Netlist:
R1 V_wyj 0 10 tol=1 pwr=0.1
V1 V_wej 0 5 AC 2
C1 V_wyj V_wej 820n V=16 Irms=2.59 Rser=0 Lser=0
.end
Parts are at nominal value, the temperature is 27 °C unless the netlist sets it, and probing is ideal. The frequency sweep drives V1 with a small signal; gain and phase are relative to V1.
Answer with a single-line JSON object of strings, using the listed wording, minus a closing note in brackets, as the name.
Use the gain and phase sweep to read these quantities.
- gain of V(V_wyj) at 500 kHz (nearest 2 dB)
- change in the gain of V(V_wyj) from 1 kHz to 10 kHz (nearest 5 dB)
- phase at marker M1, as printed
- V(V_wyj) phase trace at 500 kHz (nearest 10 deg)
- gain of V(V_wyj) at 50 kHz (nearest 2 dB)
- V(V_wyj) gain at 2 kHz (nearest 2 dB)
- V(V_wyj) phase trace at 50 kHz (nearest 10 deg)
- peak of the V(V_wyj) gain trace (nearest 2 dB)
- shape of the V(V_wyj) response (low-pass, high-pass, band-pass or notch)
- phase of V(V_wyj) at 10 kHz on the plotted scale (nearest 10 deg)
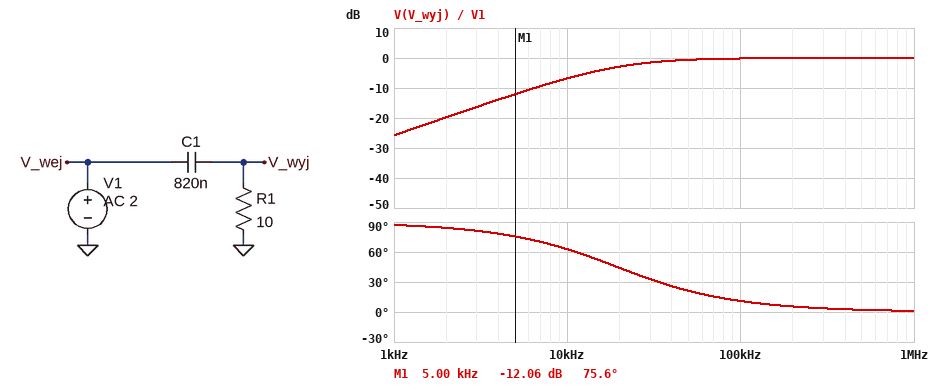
{"gain of V(V_wyj) at 500 kHz": "0 dB", "change in the gain of V(V_wyj) from 1 kHz to 10 kHz": "20 dB", "phase at marker M1, as printed": "75.6 deg", "V(V_wyj) phase trace at 500 kHz": "0 deg", "gain of V(V_wyj) at 50 kHz": "0 dB", "V(V_wyj) gain at 2 kHz": "-20 dB", "V(V_wyj) phase trace at 50 kHz": "20 deg", "peak of the V(V_wyj) gain trace": "0 dB", "shape of the V(V_wyj) response": "high-pass", "phase of V(V_wyj) at 10 kHz on the plotted scale": "60 deg"}
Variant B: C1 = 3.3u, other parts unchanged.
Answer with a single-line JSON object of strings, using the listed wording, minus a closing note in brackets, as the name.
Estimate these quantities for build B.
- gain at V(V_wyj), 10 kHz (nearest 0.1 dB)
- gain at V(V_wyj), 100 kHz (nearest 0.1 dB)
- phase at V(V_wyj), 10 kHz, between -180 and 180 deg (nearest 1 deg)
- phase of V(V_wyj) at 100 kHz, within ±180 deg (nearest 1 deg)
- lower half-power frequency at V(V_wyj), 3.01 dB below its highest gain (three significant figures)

{"gain at V(V_wyj), 10 kHz": "-0.9 dB", "gain at V(V_wyj), 100 kHz": "0 dB", "phase at V(V_wyj), 10 kHz, between -180 and 180 deg": "26 deg", "phase of V(V_wyj) at 100 kHz, within ±180 deg": "3 deg", "lower half-power frequency at V(V_wyj), 3.01 dB below its highest gain": "4.82 kHz"}
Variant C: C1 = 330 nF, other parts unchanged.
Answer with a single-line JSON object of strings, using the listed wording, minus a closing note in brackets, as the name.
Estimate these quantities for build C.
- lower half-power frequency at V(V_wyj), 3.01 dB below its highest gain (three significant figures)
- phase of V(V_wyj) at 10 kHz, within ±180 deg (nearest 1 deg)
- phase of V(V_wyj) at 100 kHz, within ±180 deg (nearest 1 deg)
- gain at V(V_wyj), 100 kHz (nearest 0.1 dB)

{"lower half-power frequency at V(V_wyj), 3.01 dB below its highest gain": "48.2 kHz", "phase of V(V_wyj) at 10 kHz, within ±180 deg": "78 deg", "phase of V(V_wyj) at 100 kHz, within ±180 deg": "26 deg", "gain at V(V_wyj), 100 kHz": "-0.9 dB"}
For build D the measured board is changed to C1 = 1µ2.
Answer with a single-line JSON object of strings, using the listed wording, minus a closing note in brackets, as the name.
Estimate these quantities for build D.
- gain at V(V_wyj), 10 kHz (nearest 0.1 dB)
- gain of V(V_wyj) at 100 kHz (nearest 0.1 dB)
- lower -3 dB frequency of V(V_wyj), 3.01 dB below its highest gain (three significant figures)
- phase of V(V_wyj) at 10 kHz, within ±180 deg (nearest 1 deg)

{"gain at V(V_wyj), 10 kHz": "-4.4 dB", "gain of V(V_wyj) at 100 kHz": "-0.1 dB", "lower -3 dB frequency of V(V_wyj), 3.01 dB below its highest gain": "13.3 kHz", "phase of V(V_wyj) at 10 kHz, within ±180 deg": "53 deg"}
